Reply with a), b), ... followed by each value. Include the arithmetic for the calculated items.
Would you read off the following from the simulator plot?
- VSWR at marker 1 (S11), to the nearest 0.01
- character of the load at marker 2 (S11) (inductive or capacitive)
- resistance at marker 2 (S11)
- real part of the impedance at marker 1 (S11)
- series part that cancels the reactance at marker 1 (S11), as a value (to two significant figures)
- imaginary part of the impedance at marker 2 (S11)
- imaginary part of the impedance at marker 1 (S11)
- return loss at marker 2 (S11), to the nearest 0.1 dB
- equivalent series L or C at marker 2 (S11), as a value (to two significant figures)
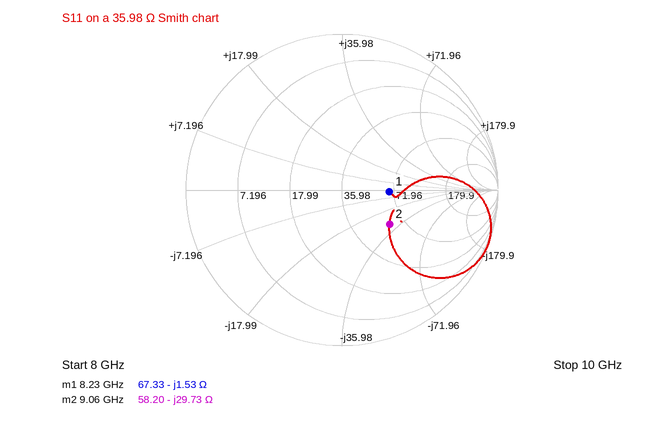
a) 1.87
b) capacitive
c) 58.20 Ω
d) 67.33 Ω
e) L = 1.53 Ω/(2π × 8.23 GHz) ≈ 30 pH
f) -29.73 Ω
g) -1.53 Ω
h) 8.5 dB
i) C = 1/(2π × 9.06 GHz × 29.73 Ω) ≈ 591 fF, so 590 fF to two significant figures
